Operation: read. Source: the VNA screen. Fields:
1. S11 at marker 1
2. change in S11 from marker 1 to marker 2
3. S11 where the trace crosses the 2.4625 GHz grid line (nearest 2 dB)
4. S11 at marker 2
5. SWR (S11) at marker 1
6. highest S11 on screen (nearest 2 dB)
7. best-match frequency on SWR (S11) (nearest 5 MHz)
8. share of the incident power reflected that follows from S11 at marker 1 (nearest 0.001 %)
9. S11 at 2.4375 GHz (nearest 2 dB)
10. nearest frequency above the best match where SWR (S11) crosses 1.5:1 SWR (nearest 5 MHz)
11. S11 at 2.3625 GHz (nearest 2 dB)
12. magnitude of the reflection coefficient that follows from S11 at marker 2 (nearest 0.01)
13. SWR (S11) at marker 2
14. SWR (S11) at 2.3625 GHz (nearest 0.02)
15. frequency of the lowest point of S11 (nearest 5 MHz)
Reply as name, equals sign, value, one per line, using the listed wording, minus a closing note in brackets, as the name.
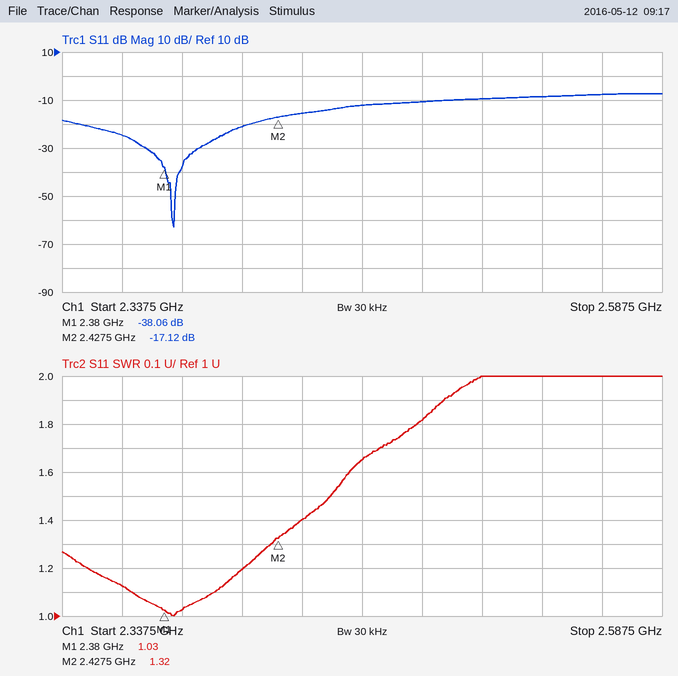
S11 at marker 1 = -38.06 dB
change in S11 from marker 1 to marker 2 = 20.94 dB
S11 where the trace crosses the 2.4625 GHz grid line = -12 dB
S11 at marker 2 = -17.12 dB
SWR (S11) at marker 1 = 1.03
highest S11 on screen = -8 dB
best-match frequency on SWR (S11) = 2.385 GHz
share of the incident power reflected that follows from S11 at marker 1 = 0.016 %
S11 at 2.4375 GHz = -16 dB
nearest frequency above the best match where SWR (S11) crosses 1.5:1 SWR = 2.450 GHz
S11 at 2.3625 GHz = -24 dB
magnitude of the reflection coefficient that follows from S11 at marker 2 = 0.14
SWR (S11) at marker 2 = 1.32
SWR (S11) at 2.3625 GHz = 1.12
frequency of the lowest point of S11 = 2.385 GHz
